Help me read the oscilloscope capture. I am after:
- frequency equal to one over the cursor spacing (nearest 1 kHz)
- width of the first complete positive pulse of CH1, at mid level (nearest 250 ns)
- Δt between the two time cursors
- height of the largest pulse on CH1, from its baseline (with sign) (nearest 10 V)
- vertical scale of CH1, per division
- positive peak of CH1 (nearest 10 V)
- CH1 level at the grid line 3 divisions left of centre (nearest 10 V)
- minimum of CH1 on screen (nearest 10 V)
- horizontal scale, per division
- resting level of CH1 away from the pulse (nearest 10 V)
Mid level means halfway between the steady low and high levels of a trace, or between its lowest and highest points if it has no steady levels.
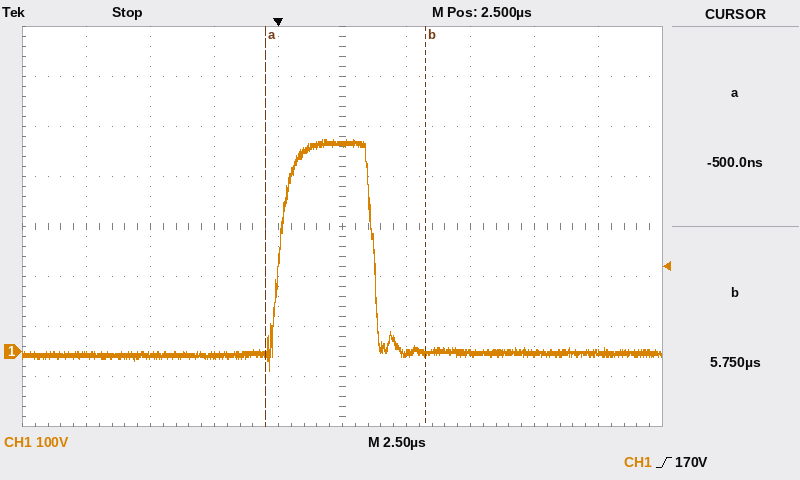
160 kHz
3.75 µs
6.25 µs
+430 V
100 V
420 V
-10 V
-40 V
2.5 µs
-10 V
